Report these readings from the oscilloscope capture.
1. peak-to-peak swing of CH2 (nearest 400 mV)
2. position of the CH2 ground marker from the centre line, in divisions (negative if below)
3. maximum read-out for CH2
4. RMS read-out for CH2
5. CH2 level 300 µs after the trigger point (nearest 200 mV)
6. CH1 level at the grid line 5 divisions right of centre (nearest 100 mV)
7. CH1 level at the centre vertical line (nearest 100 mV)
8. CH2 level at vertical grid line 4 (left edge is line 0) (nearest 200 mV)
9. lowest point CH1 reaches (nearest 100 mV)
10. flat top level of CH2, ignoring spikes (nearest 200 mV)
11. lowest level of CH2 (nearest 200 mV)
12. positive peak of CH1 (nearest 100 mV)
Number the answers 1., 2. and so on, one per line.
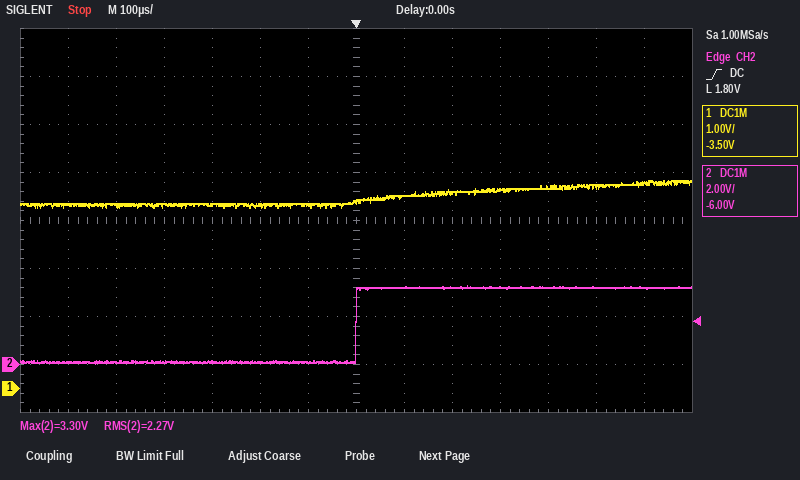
1. 3.2 V
2. -3.0 div
3. 3.30 V
4. 2.27 V
5. 3.2 V
6. 4.2 V
7. 3.9 V
8. 200 mV
9. 3.8 V
10. 3.2 V
11. 0.0 V
12. 4.3 V
